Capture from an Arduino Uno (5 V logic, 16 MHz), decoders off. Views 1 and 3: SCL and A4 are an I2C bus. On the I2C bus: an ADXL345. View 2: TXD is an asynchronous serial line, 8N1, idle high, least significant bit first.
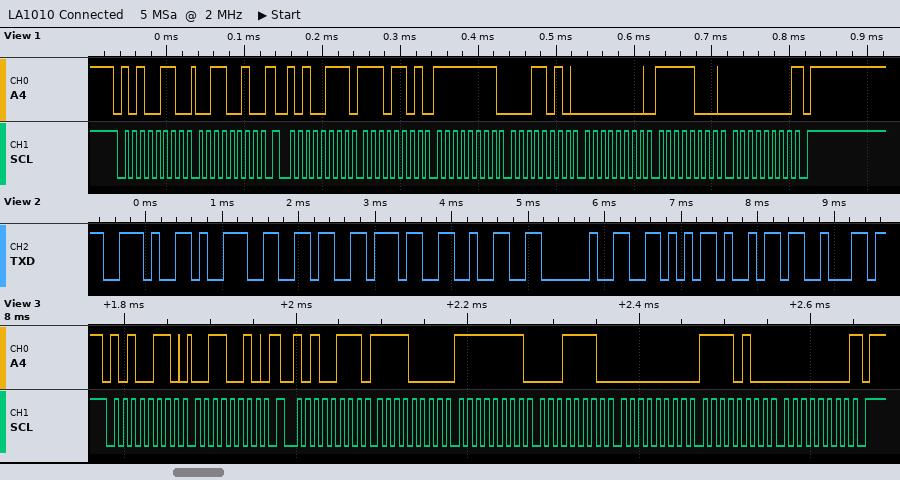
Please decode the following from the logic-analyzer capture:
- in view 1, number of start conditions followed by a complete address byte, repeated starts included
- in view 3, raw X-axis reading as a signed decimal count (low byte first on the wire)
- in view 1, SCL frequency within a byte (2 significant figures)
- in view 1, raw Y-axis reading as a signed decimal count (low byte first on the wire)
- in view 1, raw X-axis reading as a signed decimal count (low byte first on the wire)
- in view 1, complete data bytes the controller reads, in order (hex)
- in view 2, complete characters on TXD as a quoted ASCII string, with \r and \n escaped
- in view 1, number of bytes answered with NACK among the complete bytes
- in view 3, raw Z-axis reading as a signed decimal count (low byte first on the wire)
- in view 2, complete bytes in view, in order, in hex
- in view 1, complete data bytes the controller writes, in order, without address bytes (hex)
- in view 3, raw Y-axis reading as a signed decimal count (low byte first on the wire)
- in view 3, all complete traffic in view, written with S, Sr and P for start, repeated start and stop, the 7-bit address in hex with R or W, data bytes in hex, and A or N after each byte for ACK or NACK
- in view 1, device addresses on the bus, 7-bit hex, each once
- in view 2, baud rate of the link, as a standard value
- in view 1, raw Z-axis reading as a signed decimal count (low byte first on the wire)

2
-16
100 kHz
26
-19
ED FF 1A 00 F8 00
".9672 Vib"
1
244
0x2E 0x39 0x36 0x37 0x32 0x20 0x56 0x69 0x62
32
30
S 53W A 32 A Sr 53R A F0 A FF A 1E A 00 A F4 A 00 N P
0x53
9600 baud
248
